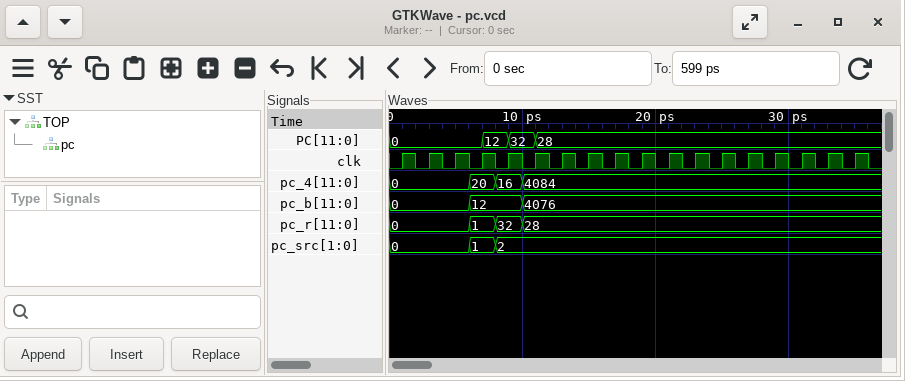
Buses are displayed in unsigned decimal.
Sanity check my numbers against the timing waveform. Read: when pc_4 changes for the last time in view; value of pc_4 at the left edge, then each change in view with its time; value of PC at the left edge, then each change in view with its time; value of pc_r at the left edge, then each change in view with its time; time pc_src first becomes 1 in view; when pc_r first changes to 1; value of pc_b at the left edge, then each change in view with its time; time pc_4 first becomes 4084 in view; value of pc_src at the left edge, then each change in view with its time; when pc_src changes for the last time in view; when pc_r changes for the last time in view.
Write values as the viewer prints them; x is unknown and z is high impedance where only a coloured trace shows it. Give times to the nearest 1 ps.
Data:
10 ps
0, 20 at 6 ps, 16 at 8 ps, 4084 at 10 ps
0, 12 at 7 ps, 32 at 9 ps, 28 at 11 ps
0, 1 at 6 ps, 32 at 8 ps, 28 at 10 ps
6 ps
6 ps
0, 12 at 6 ps, 4076 at 10 ps
10 ps
0, 1 at 6 ps, 2 at 8 ps
8 ps
10 ps
